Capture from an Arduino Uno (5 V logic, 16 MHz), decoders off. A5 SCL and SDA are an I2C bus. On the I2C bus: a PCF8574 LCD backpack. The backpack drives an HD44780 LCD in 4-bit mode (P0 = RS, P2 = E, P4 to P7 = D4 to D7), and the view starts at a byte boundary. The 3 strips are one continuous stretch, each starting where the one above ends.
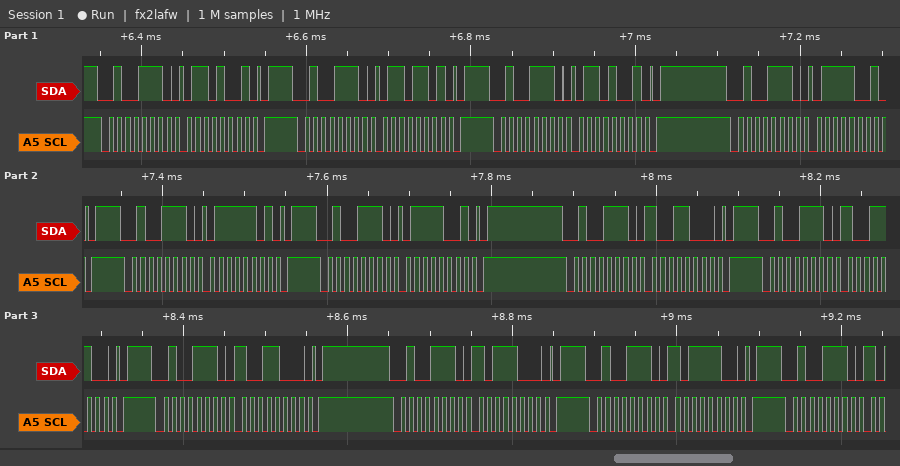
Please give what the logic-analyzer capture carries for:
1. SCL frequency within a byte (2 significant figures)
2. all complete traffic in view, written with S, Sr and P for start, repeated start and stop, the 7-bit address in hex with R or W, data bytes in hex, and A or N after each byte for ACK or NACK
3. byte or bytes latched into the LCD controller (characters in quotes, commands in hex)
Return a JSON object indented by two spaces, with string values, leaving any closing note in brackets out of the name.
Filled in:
{
  "SCL frequency within a byte": "100 kHz",
  "all complete traffic in view, written with S, Sr and P for start, repeated start and stop, the 7-bit address in hex with R or W, data bytes in hex, and A or N after each byte for ACK or NACK": "S 27W A 69 A P S 27W A 6D A P S 27W A 69 A P S 27W A 79 A P S 27W A 7D A P S 27W A 79 A P S 27W A 98 A P S 27W A 9C A P S 27W A 98 A P S 27W A B8 A P S 27W A BC A P S 27W A",
  "byte or bytes latched into the LCD controller": "'g'"
}
